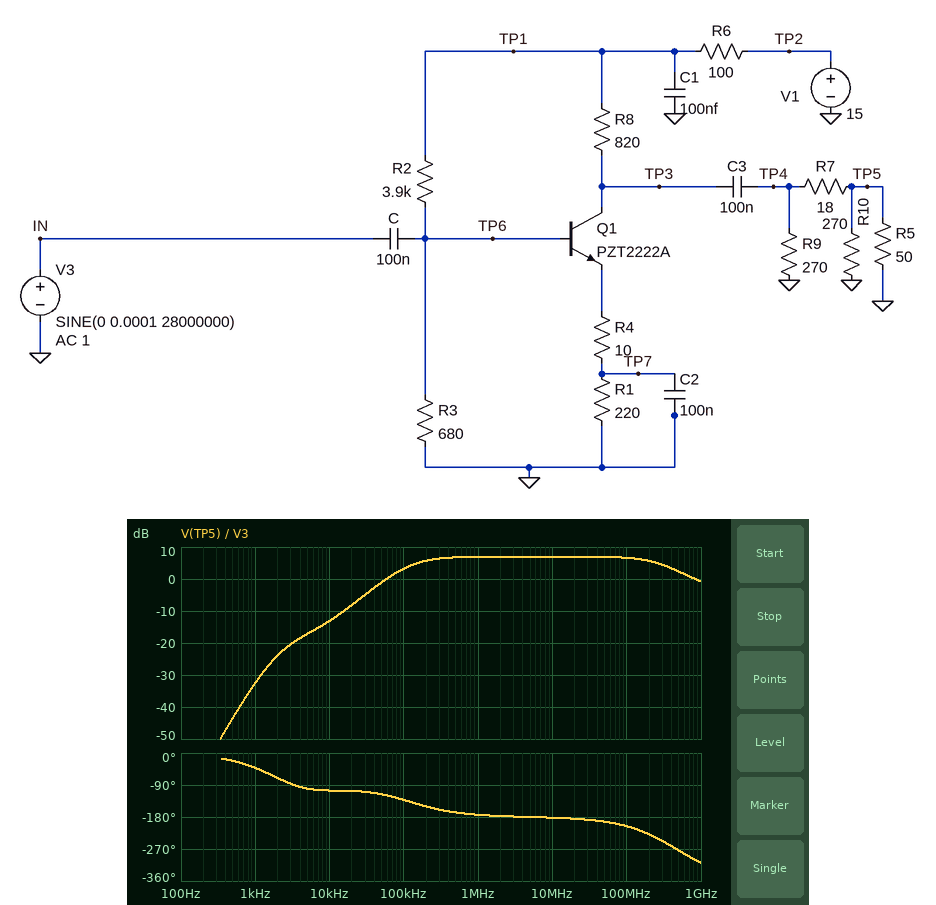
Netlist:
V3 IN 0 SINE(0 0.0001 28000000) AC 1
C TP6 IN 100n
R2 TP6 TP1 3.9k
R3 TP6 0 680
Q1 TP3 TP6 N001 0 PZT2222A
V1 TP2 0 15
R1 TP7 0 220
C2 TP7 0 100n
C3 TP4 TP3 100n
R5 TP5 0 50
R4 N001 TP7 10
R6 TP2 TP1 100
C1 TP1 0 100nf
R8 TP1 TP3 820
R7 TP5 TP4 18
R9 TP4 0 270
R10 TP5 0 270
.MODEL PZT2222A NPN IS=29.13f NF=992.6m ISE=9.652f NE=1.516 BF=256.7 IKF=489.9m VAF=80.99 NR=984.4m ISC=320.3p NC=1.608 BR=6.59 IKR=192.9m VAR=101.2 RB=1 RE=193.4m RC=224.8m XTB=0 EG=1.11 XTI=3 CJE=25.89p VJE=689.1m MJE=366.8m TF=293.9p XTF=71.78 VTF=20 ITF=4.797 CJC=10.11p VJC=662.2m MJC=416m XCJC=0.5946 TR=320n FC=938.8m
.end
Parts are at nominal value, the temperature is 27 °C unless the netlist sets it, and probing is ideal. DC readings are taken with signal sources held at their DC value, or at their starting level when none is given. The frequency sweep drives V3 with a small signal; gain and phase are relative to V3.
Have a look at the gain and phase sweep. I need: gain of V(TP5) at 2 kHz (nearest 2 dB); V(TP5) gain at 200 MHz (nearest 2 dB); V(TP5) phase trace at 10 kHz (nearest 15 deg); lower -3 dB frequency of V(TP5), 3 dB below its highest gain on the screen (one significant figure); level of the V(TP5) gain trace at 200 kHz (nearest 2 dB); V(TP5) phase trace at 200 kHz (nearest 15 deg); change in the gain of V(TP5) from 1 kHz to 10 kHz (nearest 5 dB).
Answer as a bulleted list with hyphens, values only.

- -24 dB
- 6 dB
- -105 deg
- 100 kHz
- 6 dB
- -150 deg
- 20 dB
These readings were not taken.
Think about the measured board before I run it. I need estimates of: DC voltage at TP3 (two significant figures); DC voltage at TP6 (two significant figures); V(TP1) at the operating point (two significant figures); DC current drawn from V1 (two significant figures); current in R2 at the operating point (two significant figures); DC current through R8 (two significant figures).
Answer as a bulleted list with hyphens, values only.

- 9.1 V
- 2.1 V
- 14 V
- 9.2 mA
- 3.1 mA
- 6.1 mA
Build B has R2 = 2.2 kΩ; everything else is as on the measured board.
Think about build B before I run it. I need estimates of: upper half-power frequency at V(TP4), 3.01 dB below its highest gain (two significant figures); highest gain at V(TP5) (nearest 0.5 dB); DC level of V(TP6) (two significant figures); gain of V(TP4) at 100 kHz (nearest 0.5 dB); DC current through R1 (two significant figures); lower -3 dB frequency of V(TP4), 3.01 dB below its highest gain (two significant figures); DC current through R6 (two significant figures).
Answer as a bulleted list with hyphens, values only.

- 330 MHz
- 8.0 dB
- 3.2 V
- 7.0 dB
- 11 mA
- 130 kHz
- 15 mA
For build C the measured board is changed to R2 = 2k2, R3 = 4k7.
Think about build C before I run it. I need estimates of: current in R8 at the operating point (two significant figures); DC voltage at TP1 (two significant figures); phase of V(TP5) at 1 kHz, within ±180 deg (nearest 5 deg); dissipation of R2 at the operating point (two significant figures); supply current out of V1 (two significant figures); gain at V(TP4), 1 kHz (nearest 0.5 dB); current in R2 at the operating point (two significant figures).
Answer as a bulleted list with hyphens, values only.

- 12 mA
- 13 V
- 160 deg
- 38 mW
- 16 mA
- -50.5 dB
- 4.2 mA
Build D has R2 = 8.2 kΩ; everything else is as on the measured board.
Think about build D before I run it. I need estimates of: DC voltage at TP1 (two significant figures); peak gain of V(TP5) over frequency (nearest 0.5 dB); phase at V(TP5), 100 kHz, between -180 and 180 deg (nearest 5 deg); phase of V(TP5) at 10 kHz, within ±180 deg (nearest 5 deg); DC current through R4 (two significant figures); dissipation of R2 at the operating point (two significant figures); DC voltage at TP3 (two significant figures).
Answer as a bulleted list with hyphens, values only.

- 15 V
- 3.0 dB
- -145 deg
- -110 deg
- 2.1 mA
- 22 mW
- 13 V
